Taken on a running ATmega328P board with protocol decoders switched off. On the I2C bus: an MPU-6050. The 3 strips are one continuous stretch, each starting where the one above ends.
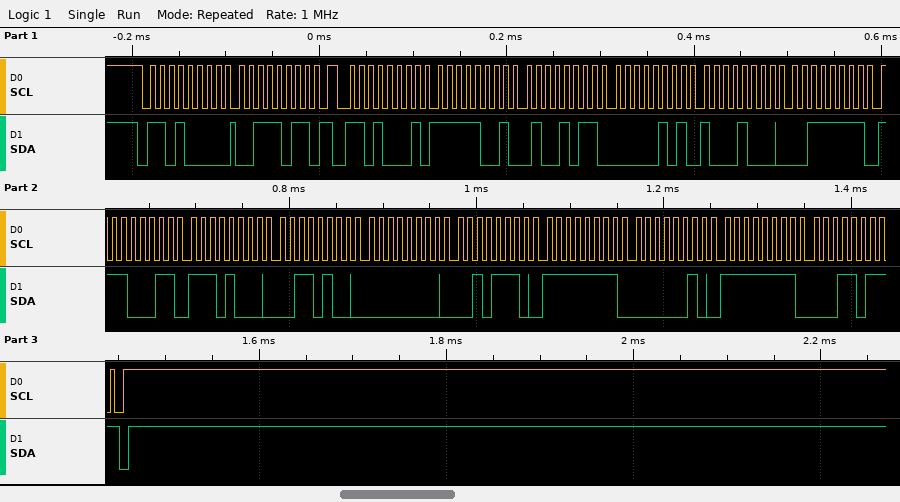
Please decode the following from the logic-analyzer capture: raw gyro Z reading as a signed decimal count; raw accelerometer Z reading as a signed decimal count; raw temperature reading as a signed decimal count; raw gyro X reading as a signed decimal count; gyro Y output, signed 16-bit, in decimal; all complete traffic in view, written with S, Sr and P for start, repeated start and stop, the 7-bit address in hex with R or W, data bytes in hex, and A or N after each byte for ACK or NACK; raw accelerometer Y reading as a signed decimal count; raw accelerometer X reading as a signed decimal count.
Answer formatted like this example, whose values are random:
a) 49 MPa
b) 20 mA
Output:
a) -229
b) 16355
c) -6092
d) 46
e) -254
f) S 68W A 3B A Sr 68R A F9 A 4B A 05 A 88 A 3F A E3 A E8 A 34 A 00 A 2E A FF A 02 A FF A 1B N P
g) 1416
h) -1717
